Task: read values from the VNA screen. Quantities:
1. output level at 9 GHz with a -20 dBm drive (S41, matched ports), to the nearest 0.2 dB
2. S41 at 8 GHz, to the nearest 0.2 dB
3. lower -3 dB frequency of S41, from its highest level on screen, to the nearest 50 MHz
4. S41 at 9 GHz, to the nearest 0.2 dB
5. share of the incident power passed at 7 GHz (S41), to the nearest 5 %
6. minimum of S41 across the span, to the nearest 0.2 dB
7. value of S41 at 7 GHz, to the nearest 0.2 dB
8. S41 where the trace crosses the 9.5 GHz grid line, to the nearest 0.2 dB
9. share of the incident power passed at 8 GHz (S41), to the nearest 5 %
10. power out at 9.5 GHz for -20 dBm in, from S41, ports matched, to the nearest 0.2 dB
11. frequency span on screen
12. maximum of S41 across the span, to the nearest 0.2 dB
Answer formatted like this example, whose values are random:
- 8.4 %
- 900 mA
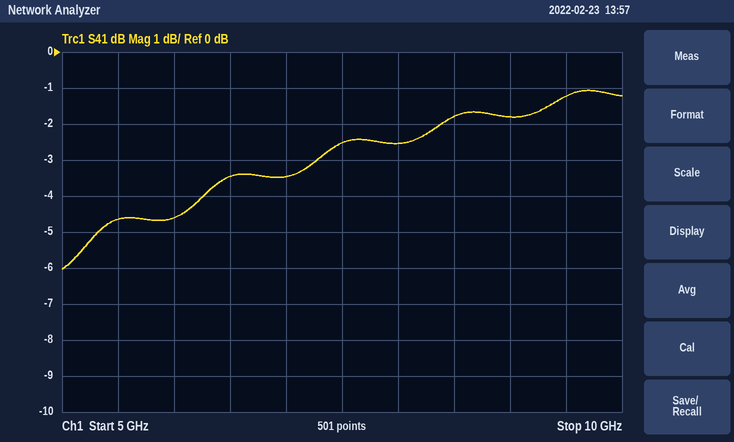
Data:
- -21.8 dBm
- -2.6 dB
- 6.25 GHz
- -1.8 dB
- 45 %
- -6.0 dB
- -3.4 dB
- -1.2 dB
- 55 %
- -21.2 dBm
- 5 GHz
- -1.0 dB
